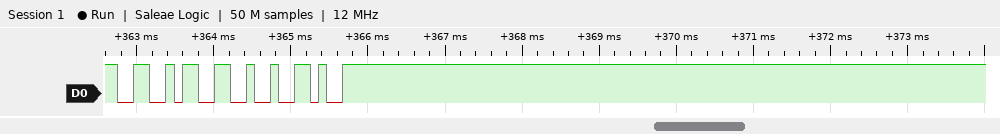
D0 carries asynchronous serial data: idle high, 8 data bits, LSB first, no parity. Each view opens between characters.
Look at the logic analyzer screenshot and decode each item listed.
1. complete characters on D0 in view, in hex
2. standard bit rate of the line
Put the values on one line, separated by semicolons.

A6, 26, 96; 9600 baud
